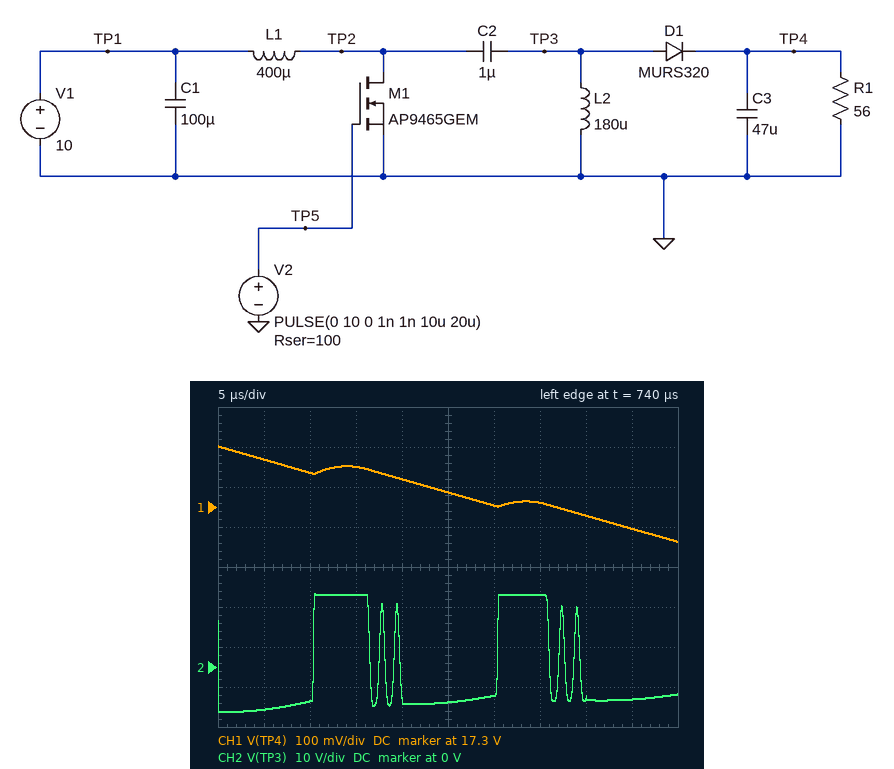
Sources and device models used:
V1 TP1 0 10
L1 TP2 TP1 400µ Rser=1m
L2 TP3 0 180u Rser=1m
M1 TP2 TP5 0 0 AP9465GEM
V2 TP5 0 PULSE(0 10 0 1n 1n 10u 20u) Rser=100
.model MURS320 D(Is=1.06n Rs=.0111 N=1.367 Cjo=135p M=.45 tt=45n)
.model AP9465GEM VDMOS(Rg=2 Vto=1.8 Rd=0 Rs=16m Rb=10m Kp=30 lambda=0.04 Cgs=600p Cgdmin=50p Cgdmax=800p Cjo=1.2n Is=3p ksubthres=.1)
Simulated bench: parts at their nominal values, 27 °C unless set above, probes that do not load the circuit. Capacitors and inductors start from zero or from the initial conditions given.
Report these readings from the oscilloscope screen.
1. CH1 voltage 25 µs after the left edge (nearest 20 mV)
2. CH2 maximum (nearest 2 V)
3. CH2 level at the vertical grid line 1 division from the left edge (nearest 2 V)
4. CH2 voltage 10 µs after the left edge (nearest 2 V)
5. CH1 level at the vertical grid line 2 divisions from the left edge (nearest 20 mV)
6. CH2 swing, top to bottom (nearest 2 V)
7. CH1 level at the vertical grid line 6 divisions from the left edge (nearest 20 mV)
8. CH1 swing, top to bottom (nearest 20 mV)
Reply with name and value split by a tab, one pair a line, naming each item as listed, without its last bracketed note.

CH1 voltage 25 µs after the left edge	17.34 V
CH2 maximum	18 V
CH2 level at the vertical grid line 1 division from the left edge	-10 V
CH2 voltage 10 µs after the left edge	-8 V
CH1 level at the vertical grid line 2 divisions from the left edge	17.38 V
CH2 swing, top to bottom	30 V
CH1 level at the vertical grid line 6 divisions from the left edge	17.30 V
CH1 swing, top to bottom	240 mV
